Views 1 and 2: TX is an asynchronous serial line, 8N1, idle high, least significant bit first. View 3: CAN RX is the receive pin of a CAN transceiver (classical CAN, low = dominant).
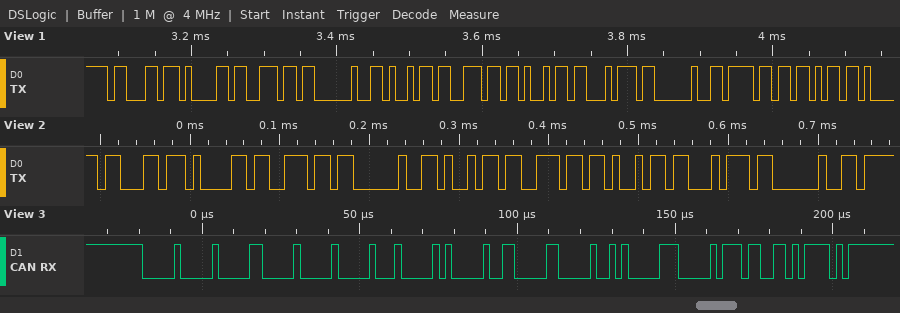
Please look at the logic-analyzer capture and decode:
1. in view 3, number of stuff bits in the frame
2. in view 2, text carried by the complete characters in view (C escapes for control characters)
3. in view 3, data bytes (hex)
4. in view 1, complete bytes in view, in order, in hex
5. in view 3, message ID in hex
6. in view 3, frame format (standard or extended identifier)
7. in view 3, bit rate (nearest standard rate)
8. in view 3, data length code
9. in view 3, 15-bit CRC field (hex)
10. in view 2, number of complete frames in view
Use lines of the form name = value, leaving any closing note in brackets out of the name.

in view 3, number of stuff bits in the frame = 12
in view 2, text carried by the complete characters in view = "can init "
in view 3, data bytes = 00 01 02 03 04 05 06 07
in view 1, complete bytes in view, in order, in hex = 63 61 6E 20 69 6E 69 74 20 6F 6B
in view 3, message ID in hex = 0x000
in view 3, frame format = standard
in view 3, bit rate = 500 kbit/s
in view 3, data length code = 8
in view 3, 15-bit CRC field = 0x335E
in view 2, number of complete frames in view = 9
